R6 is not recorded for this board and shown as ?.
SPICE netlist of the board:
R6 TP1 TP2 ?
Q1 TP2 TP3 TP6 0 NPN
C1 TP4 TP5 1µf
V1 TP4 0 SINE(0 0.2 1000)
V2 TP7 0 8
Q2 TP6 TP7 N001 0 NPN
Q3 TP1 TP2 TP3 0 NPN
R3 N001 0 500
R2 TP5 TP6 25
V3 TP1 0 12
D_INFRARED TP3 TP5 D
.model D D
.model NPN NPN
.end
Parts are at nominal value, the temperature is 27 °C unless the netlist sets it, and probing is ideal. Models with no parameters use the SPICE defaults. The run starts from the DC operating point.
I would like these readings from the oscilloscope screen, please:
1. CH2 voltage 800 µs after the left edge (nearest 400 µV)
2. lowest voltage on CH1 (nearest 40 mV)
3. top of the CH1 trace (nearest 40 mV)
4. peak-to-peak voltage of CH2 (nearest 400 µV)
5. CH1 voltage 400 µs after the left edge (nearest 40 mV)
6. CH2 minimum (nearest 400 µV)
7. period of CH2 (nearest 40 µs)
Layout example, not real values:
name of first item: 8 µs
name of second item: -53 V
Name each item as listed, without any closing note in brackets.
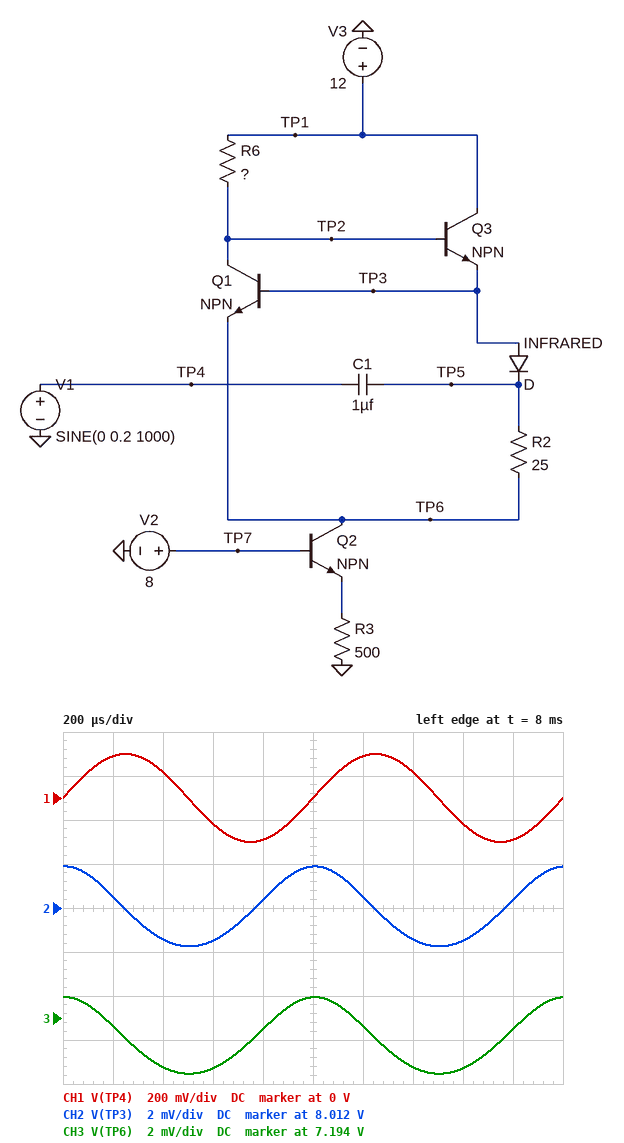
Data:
CH2 voltage 800 µs after the left edge: 8.0124 V
lowest voltage on CH1: -200 mV
top of the CH1 trace: 200 mV
peak-to-peak voltage of CH2: 3.6 mV
CH1 voltage 400 µs after the left edge: 120 mV
CH2 minimum: 8.0104 V
period of CH2: 1.00 ms
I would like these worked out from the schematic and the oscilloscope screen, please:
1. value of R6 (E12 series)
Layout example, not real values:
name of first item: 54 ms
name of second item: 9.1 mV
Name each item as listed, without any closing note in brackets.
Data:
value of R6: 560 Ω
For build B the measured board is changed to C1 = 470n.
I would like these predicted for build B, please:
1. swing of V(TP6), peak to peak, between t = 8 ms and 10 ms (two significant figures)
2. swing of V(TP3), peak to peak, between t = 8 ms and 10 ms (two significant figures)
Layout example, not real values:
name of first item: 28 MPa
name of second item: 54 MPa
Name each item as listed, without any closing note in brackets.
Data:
swing of V(TP6), peak to peak, between t = 8 ms and 10 ms: 1.6 mV
swing of V(TP3), peak to peak, between t = 8 ms and 10 ms: 1.7 mV
